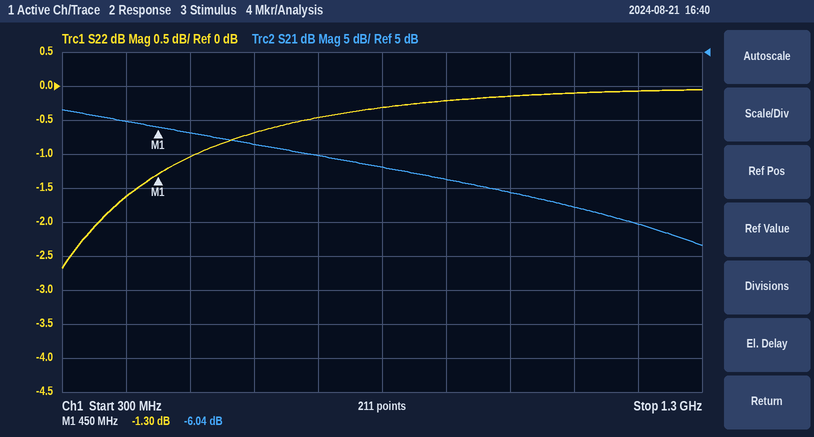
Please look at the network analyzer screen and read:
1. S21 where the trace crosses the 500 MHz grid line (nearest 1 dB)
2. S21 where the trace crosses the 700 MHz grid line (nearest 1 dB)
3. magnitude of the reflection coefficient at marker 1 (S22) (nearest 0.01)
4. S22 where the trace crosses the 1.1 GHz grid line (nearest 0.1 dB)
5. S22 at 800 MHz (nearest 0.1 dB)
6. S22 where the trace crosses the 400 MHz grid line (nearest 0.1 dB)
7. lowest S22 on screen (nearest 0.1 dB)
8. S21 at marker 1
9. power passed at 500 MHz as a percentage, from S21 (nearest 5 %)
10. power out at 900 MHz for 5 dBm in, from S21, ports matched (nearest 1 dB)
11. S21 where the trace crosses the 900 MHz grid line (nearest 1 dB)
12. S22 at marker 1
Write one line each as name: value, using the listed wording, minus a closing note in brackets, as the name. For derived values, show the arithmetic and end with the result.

S21 where the trace crosses the 500 MHz grid line: -7 dB
S21 where the trace crosses the 700 MHz grid line: -10 dB
magnitude of the reflection coefficient at marker 1 (S22): 10^(-1.3/20) ≈ 0.86
S22 where the trace crosses the 1.1 GHz grid line: -0.1 dB
S22 at 800 MHz: -0.3 dB
S22 where the trace crosses the 400 MHz grid line: -1.6 dB
lowest S22 on screen: -2.7 dB
S21 at marker 1: -6.04 dB
power passed at 500 MHz as a percentage, from S21: 10^(-7/10) ≈ 20 %
power out at 900 MHz for 5 dBm in, from S21, ports matched: 5 dBm + (-14 dB) = -9 dBm
S21 where the trace crosses the 900 MHz grid line: -14 dB
S22 at marker 1: -1.30 dB
